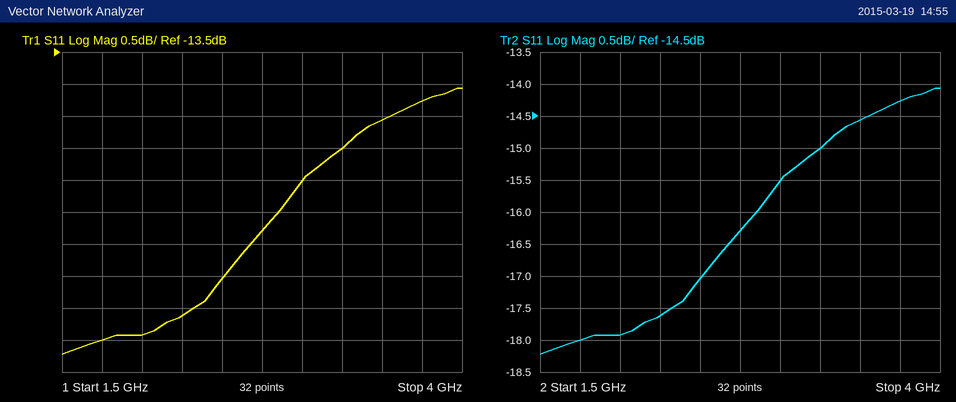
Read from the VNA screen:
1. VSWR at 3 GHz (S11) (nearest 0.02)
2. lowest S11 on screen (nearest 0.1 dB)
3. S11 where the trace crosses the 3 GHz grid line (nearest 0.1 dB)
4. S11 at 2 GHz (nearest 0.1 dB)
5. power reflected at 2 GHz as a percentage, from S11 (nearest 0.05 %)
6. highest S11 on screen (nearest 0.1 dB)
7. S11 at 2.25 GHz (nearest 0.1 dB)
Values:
1.40
-18.2 dB
-15.5 dB
-17.9 dB
1.60 %
-14.1 dB
-17.6 dB
